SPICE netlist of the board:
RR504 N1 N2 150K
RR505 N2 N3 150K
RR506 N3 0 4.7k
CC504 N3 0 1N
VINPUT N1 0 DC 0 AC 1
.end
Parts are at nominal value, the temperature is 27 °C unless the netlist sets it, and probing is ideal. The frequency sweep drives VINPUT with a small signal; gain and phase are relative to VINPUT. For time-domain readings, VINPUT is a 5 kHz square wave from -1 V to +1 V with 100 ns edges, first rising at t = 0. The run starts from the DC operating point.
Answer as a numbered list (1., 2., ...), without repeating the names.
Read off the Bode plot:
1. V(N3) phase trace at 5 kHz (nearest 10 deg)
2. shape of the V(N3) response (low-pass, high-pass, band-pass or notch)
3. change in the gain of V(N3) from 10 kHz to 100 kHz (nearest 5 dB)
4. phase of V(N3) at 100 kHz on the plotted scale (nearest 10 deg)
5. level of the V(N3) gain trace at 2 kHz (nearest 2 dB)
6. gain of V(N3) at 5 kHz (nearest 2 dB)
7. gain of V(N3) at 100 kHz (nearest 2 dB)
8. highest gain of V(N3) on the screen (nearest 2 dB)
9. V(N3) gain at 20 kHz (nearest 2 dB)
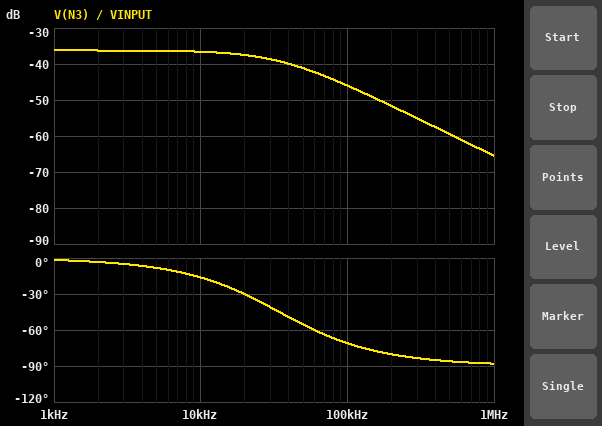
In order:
1. -10 deg
2. low-pass
3. -10 dB
4. -70 deg
5. -36 dB
6. -36 dB
7. -46 dB
8. -36 dB
9. -38 dB
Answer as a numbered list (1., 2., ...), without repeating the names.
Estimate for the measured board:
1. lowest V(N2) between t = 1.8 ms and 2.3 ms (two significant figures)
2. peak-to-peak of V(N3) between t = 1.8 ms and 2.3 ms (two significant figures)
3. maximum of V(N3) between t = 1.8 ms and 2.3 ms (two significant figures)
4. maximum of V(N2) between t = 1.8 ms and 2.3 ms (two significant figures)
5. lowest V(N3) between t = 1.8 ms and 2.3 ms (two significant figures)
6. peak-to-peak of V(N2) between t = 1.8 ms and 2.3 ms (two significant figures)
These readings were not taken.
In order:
1. -510 mV
2. 31 mV
3. 15 mV
4. 510 mV
5. -15 mV
6. 1.0 V
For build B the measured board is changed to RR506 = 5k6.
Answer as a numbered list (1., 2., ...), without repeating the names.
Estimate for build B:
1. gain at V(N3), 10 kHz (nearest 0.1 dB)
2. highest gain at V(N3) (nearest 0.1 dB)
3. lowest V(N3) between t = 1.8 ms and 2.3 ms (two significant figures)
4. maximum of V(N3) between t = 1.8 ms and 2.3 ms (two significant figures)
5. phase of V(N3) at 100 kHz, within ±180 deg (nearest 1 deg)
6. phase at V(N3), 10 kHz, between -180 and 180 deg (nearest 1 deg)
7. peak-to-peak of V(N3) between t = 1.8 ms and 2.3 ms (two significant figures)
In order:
1. -35.2 dB
2. -34.7 dB
3. -18 mV
4. 18 mV
5. -74 deg
6. -19 deg
7. 37 mV
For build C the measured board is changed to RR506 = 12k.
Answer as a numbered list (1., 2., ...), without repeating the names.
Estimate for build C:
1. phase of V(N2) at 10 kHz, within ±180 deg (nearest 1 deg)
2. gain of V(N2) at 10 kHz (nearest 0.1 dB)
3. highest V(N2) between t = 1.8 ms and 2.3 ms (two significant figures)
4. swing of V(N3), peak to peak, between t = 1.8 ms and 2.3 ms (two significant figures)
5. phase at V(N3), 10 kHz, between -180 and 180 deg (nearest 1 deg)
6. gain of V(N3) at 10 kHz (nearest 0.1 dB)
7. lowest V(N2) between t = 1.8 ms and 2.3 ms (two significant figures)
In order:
1. -1 deg
2. -5.8 dB
3. 520 mV
4. 77 mV
5. -36 deg
6. -30.1 dB
7. -520 mV
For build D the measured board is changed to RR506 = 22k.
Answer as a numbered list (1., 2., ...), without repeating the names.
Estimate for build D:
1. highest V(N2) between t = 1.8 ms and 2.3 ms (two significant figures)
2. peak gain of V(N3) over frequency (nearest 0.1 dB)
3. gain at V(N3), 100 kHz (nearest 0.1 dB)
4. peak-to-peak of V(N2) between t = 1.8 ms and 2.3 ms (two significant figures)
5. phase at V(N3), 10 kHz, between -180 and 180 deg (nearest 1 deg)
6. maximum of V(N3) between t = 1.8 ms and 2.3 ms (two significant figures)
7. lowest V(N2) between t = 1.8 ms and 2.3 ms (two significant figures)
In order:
1. 530 mV
2. -23.3 dB
3. -45.5 dB
4. 1.1 V
5. -52 deg
6. 67 mV
7. -530 mV
